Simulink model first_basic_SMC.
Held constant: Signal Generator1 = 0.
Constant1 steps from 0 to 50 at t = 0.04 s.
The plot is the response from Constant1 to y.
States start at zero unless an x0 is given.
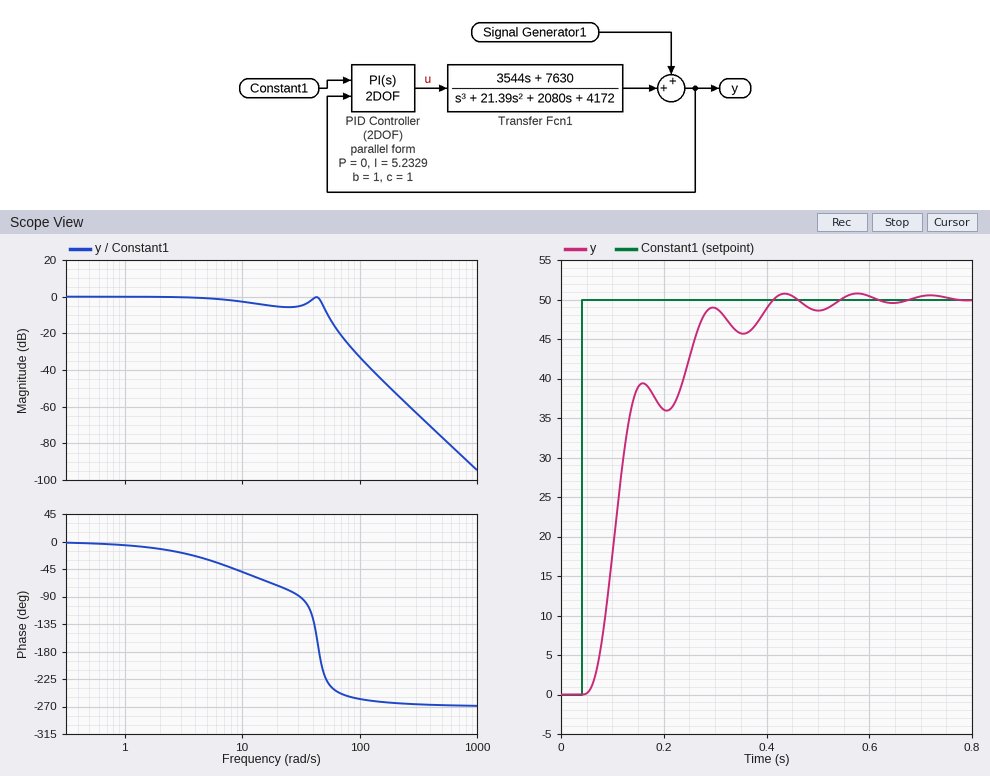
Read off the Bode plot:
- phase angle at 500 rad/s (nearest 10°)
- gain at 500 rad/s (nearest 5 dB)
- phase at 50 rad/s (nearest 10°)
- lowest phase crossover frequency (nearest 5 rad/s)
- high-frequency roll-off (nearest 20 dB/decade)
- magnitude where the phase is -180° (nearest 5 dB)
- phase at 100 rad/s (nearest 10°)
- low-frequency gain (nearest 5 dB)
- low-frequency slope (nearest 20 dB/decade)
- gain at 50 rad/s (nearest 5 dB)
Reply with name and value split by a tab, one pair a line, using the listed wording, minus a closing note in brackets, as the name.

phase angle at 500 rad/s	-270°
gain at 500 rad/s	-75 dB
phase at 50 rad/s	-220°
lowest phase crossover frequency	45 rad/s
high-frequency roll-off	-60 dB/decade
magnitude where the phase is -180°	0 dB
phase at 100 rad/s	-260°
low-frequency gain	0 dB
low-frequency slope	0 dB/decade
gain at 50 rad/s	-5 dB
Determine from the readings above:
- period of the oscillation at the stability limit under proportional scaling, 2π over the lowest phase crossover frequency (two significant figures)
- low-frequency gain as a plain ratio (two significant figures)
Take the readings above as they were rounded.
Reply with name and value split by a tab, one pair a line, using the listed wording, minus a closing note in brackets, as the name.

period of the oscillation at the stability limit under proportional scaling, 2π over the lowest phase crossover frequency	0.14 s
low-frequency gain as a plain ratio	1.0
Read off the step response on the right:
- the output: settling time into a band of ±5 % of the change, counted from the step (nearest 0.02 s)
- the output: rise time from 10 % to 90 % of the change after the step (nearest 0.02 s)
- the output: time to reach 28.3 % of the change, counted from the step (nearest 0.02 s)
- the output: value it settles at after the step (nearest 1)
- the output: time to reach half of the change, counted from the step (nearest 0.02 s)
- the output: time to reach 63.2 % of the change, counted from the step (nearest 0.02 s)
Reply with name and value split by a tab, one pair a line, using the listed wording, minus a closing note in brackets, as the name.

the output: settling time into a band of ±5 % of the change, counted from the step	0.34 s
the output: rise time from 10 % to 90 % of the change after the step	0.18 s
the output: time to reach 28.3 % of the change, counted from the step	0.06 s
the output: value it settles at after the step	50
the output: time to reach half of the change, counted from the step	0.08 s
the output: time to reach 63.2 % of the change, counted from the step	0.08 s
